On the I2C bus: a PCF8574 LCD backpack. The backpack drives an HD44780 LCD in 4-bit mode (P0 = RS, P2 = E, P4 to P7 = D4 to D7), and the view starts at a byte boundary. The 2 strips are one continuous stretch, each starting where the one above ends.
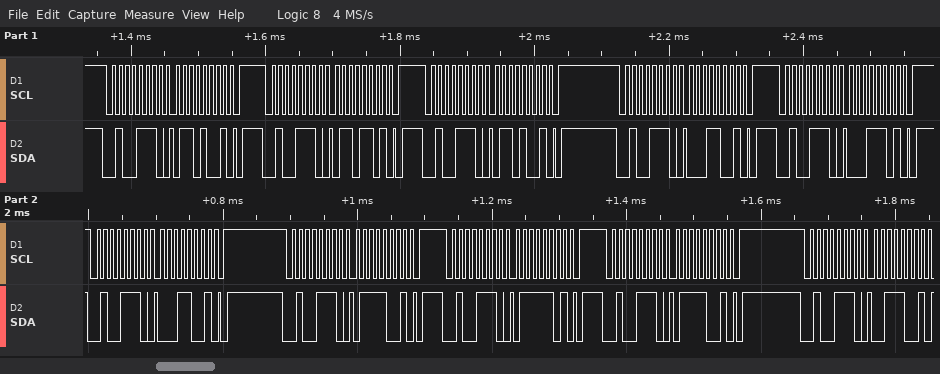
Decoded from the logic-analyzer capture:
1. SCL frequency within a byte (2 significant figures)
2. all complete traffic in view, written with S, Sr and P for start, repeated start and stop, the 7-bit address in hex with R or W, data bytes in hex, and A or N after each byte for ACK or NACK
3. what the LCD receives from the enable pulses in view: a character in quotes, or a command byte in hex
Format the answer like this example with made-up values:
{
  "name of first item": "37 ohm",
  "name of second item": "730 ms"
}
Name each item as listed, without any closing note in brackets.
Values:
{
  "SCL frequency within a byte": "100 kHz",
  "all complete traffic in view, written with S, Sr and P for start, repeated start and stop, the 7-bit address in hex with R or W, data bytes in hex, and A or N after each byte for ACK or NACK": "S 27W A 69 A P S 27W A 6D A P S 27W A 69 A P S 27W A 19 A P S 27W A 1D A P S 27W A 19 A P S 27W A 79 A P S 27W A 7D A P S 27W A 79 A P S 27W A 39 A",
  "what the LCD receives from the enable pulses in view: a character in quotes, or a command byte in hex": "'a'"
}
